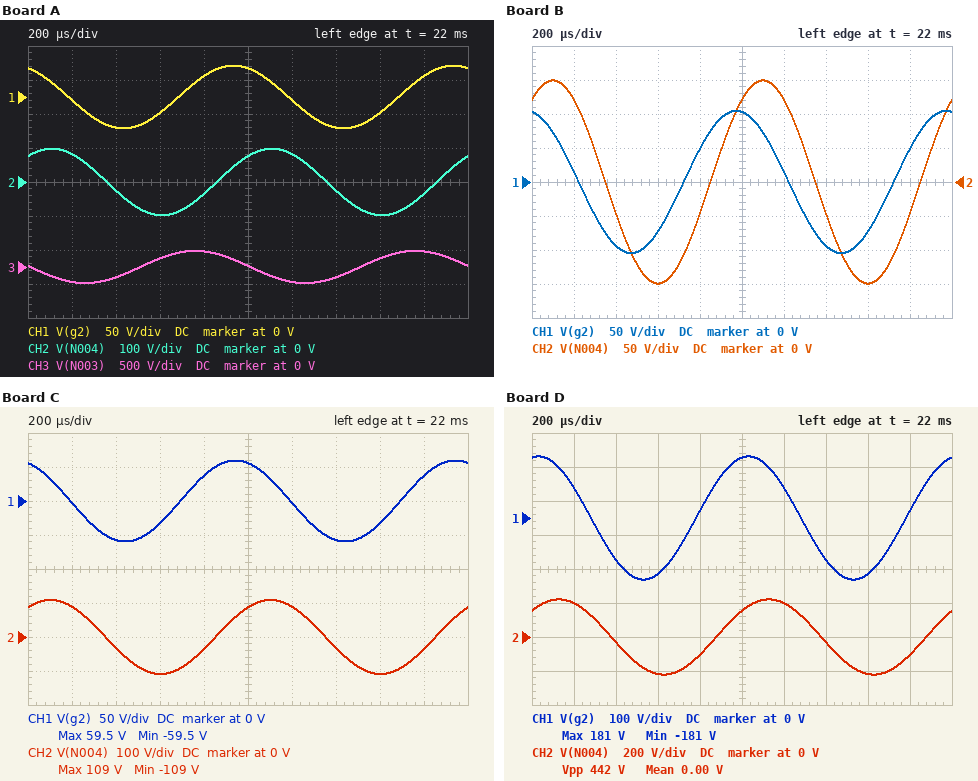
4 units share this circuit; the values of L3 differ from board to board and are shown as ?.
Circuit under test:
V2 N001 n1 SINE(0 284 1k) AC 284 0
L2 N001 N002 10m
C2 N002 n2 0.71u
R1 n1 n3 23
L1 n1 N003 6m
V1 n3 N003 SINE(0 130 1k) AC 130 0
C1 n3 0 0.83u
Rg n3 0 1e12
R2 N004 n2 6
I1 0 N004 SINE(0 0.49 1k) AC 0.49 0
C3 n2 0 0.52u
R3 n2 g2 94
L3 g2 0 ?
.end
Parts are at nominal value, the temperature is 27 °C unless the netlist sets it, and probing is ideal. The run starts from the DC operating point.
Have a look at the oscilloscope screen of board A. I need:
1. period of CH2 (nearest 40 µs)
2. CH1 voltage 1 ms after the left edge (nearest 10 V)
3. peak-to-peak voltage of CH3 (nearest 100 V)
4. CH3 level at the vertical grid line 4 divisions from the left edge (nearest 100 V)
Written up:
1.00 ms
40 V
500 V
200 V
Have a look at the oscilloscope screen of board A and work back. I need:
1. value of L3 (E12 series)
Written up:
8.2 mH
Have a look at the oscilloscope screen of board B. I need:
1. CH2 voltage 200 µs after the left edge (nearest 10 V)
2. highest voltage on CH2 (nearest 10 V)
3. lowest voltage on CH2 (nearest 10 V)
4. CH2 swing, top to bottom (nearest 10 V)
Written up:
120 V
150 V
-150 V
300 V
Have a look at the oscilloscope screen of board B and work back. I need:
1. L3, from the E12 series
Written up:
15 mH
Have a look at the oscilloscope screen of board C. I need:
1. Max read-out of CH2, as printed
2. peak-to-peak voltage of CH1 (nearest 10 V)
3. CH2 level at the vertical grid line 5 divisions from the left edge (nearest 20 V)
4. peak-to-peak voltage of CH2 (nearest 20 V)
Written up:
109 V
120 V
80 V
220 V
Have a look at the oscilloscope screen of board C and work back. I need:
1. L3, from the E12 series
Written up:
10 mH
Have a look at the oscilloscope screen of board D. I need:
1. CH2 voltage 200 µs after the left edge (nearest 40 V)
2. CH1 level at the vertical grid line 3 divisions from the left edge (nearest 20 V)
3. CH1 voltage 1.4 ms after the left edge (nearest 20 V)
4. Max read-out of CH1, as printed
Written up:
200 V
-160 V
-120 V
181 V
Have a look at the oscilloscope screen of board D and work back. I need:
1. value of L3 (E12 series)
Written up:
22 mH
